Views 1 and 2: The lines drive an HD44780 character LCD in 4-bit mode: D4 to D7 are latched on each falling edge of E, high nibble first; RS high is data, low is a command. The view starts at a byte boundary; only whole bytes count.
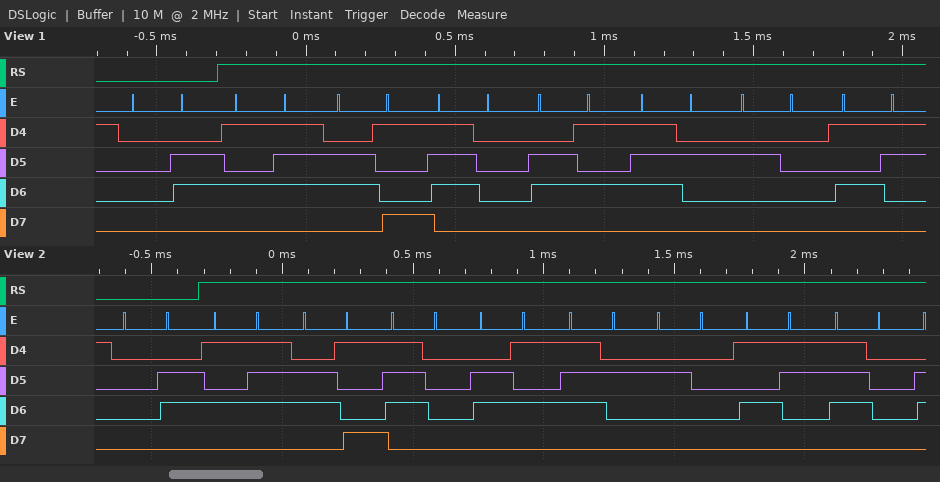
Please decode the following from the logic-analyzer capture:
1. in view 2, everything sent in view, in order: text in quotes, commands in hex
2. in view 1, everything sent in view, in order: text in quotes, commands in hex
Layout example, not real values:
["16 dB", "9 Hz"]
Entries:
["0x06 \"Wiper Sp\"", "0x06 \"Wiper S\""]
